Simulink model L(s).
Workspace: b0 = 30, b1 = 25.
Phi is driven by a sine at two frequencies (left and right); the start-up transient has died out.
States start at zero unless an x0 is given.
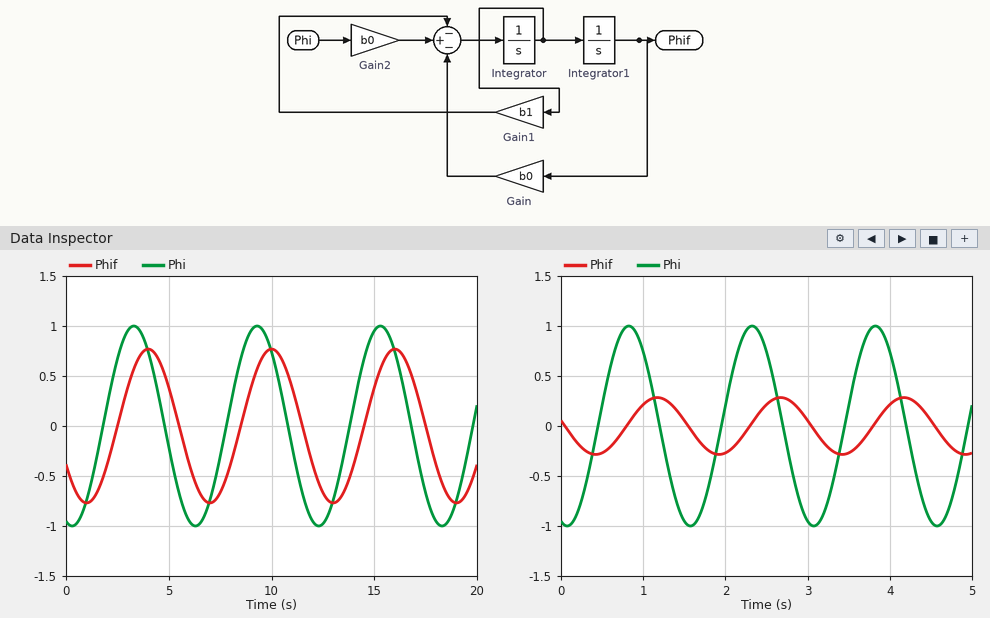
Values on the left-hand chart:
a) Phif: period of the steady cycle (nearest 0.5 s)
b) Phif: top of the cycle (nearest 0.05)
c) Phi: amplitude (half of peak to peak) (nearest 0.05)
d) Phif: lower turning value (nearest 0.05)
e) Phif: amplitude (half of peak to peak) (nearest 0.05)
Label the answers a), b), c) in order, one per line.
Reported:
a) 6.0 s
b) 0.75
c) 1.00
d) -0.75
e) 0.75
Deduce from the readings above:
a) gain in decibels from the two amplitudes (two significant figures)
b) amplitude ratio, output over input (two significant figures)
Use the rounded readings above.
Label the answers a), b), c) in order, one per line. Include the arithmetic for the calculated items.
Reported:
a) 20 log10(0.75 / 1) = -2.5 dB
b) 0.75 / 1 = 0.75
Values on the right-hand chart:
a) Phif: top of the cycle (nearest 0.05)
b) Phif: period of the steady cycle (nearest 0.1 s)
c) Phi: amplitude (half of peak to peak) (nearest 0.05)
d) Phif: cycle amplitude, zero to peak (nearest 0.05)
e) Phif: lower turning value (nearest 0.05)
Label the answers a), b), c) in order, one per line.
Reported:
a) 0.30
b) 1.5 s
c) 1.00
d) 0.30
e) -0.30
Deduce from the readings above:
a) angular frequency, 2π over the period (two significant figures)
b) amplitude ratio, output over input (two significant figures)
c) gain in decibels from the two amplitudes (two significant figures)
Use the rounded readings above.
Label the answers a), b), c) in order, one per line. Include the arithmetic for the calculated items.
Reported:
a) 2π / 1.5 = 4.2 rad/s
b) 0.3 / 1 = 0.30
c) 20 log10(0.3 / 1) = -10 dB
